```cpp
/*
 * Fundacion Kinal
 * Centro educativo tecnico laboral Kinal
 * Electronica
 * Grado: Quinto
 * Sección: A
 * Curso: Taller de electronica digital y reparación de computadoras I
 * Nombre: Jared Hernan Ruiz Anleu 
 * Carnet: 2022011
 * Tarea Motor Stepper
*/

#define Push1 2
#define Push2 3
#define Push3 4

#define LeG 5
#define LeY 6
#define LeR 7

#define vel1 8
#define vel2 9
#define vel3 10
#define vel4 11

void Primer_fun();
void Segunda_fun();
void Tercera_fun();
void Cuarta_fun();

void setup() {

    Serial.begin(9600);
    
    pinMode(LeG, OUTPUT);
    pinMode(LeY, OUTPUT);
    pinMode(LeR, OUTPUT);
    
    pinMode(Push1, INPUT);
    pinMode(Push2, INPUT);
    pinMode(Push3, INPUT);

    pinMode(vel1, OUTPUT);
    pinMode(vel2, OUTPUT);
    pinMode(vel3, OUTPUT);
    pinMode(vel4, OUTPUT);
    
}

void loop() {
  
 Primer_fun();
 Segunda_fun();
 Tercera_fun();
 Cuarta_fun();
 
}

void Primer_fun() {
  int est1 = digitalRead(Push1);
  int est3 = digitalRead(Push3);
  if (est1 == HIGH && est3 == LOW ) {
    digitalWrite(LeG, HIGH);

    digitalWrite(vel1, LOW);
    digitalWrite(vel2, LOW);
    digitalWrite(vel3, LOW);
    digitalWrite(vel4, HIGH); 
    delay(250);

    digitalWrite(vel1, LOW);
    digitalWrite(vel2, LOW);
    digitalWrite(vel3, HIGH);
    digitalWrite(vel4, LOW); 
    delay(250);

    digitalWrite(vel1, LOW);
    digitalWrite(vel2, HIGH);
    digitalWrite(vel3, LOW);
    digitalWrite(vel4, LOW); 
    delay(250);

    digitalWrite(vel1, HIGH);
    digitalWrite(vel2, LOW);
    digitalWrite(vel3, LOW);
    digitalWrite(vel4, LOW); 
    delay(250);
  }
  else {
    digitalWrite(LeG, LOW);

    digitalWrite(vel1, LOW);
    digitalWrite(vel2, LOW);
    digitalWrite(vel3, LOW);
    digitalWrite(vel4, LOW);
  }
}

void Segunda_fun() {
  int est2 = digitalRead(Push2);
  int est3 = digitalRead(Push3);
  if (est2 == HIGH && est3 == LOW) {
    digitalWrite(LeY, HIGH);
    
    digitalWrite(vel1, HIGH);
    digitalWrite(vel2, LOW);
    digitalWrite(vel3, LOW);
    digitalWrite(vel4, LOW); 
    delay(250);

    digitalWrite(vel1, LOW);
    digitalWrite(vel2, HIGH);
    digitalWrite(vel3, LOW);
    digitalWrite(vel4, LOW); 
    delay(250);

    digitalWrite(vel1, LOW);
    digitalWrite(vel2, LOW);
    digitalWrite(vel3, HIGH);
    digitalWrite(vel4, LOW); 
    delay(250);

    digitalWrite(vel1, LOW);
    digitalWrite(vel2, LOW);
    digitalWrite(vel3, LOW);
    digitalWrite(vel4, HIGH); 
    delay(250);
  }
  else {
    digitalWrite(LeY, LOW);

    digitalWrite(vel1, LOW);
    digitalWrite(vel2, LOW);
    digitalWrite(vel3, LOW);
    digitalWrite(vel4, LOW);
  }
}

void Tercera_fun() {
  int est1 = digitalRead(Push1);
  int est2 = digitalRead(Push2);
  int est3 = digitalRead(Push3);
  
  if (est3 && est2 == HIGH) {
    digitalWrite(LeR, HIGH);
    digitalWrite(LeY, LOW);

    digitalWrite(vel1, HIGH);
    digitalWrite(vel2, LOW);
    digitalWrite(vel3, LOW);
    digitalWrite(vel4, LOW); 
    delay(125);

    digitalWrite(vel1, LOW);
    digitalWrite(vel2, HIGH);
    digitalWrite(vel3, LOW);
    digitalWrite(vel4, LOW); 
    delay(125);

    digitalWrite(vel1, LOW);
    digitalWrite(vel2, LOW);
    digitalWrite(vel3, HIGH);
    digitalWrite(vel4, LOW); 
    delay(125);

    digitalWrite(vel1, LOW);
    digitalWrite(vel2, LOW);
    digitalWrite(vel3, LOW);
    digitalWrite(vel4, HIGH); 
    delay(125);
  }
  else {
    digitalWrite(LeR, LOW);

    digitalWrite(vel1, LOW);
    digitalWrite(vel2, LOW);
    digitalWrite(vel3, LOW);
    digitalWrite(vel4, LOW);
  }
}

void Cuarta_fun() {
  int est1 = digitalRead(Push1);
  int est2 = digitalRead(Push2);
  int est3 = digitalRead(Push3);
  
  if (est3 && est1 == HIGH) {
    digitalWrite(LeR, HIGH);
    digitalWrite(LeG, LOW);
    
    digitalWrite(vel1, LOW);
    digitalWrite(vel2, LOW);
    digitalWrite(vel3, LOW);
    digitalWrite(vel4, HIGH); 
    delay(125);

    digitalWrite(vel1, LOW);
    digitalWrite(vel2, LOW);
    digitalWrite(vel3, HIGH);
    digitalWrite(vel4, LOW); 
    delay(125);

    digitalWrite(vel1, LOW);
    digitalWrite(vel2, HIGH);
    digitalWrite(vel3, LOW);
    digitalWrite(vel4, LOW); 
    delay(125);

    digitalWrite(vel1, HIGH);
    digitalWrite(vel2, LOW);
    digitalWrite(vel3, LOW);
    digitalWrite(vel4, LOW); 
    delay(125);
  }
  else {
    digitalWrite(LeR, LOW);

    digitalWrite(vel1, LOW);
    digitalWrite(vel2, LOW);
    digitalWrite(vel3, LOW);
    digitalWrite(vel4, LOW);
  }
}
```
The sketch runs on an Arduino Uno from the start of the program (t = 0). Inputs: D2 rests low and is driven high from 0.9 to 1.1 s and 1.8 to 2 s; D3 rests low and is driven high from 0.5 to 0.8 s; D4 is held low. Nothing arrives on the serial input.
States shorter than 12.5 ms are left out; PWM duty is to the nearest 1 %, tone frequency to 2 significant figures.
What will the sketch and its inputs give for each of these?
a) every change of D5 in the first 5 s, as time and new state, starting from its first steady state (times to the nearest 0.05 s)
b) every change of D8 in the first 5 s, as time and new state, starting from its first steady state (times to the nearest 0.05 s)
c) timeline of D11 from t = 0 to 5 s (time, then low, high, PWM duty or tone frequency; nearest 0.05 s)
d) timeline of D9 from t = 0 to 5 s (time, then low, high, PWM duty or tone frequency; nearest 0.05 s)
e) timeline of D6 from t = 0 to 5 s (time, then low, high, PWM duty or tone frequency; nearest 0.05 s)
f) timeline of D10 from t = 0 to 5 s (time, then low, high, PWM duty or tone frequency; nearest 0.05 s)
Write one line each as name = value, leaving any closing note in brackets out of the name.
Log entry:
every change of D5 in the first 5 s, as time and new state, starting from its first steady state = 0 s low; 1.8 s high; 2.8 s low
every change of D8 in the first 5 s, as time and new state, starting from its first steady state = 0 s low; 0.5 s high; 0.75 s low; 2.55 s high; 2.8 s low
timeline of D11 from t = 0 to 5 s = 0 s low; 1.25 s high; 1.5 s low; 1.8 s high; 2.05 s low
timeline of D9 from t = 0 to 5 s = 0 s low; 0.75 s high; 1 s low; 2.3 s high; 2.55 s low
timeline of D6 from t = 0 to 5 s = 0 s low; 0.5 s high; 1.5 s low
timeline of D10 from t = 0 to 5 s = 0 s low; 1 s high; 1.25 s low; 2.05 s high; 2.3 s low
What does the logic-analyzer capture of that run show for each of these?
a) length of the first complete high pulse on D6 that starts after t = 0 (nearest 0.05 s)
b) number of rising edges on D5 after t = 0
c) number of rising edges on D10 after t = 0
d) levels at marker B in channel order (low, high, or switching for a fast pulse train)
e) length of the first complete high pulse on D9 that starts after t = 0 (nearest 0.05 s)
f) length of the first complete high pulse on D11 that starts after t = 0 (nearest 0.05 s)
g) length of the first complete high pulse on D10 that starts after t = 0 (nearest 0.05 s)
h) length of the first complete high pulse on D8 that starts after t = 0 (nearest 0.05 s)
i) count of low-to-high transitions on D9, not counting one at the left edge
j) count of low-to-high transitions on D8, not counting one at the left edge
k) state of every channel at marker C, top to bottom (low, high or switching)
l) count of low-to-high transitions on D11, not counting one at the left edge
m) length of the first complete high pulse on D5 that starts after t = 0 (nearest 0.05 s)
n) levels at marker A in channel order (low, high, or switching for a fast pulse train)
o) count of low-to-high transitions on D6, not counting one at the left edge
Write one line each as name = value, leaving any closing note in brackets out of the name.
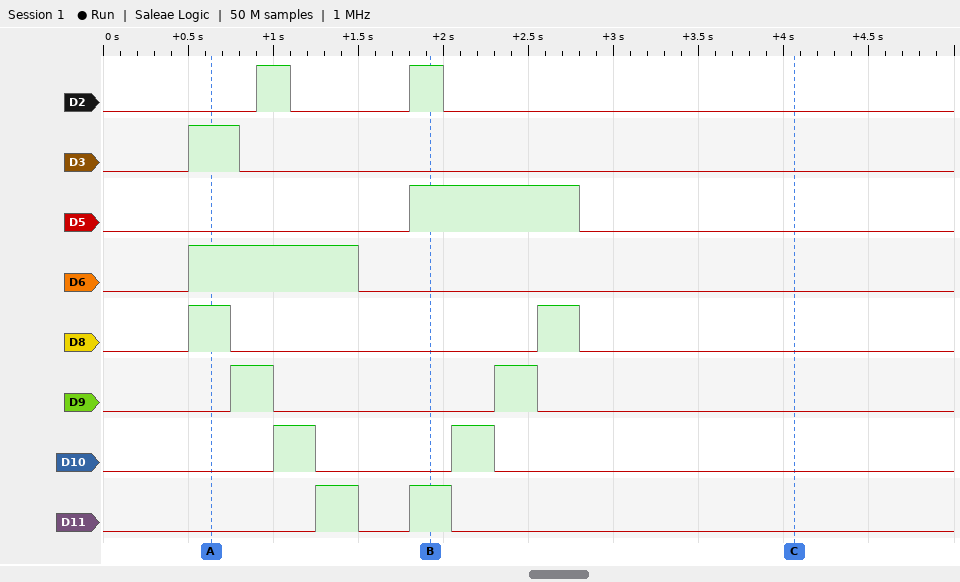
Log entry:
length of the first complete high pulse on D6 that starts after t = 0 = 1.00 s
number of rising edges on D5 after t = 0 = 1
number of rising edges on D10 after t = 0 = 2
levels at marker B in channel order = D2 high, D3 low, D5 high, D6 low, D8 low, D9 low, D10 low, D11 high
length of the first complete high pulse on D9 that starts after t = 0 = 0.25 s
length of the first complete high pulse on D11 that starts after t = 0 = 0.25 s
length of the first complete high pulse on D10 that starts after t = 0 = 0.25 s
length of the first complete high pulse on D8 that starts after t = 0 = 0.25 s
count of low-to-high transitions on D9, not counting one at the left edge = 2
count of low-to-high transitions on D8, not counting one at the left edge = 2
state of every channel at marker C, top to bottom = D2 low, D3 low, D5 low, D6 low, D8 low, D9 low, D10 low, D11 low
count of low-to-high transitions on D11, not counting one at the left edge = 2
length of the first complete high pulse on D5 that starts after t = 0 = 1.00 s
levels at marker A in channel order = D2 low, D3 high, D5 low, D6 high, D8 high, D9 low, D10 low, D11 low
count of low-to-high transitions on D6, not counting one at the left edge = 1
